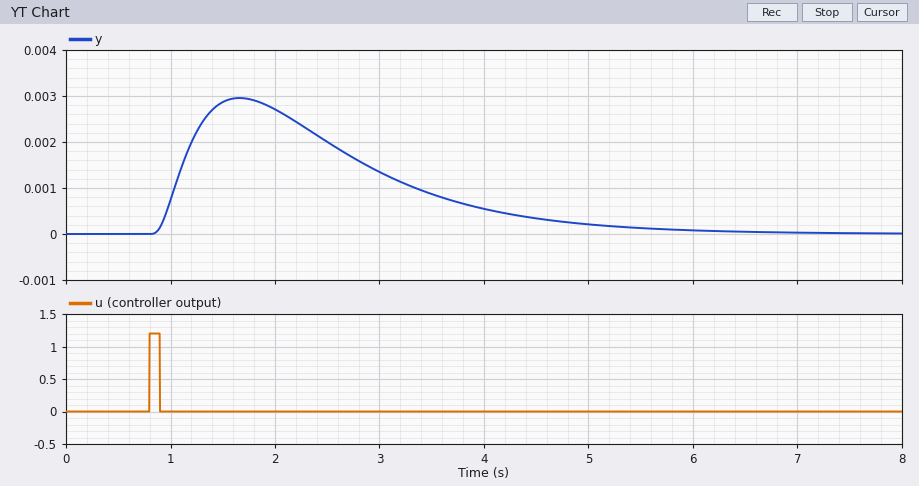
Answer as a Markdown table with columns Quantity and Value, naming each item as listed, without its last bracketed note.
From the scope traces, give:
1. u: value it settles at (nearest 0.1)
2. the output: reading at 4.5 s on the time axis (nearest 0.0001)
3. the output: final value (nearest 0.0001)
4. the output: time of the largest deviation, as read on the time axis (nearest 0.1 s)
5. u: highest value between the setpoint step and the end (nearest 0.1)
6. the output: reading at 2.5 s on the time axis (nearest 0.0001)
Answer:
| Quantity | Value |
|---|---|
| u: value it settles at | 0.0 |
| the output: reading at 4.5 s on the time axis | 0.0003 |
| the output: final value | 0.0000 |
| the output: time of the largest deviation, as read on the time axis | 1.7 s |
| u: highest value between the setpoint step and the end | 1.2 |
| the output: reading at 2.5 s on the time axis | 0.0020 |
